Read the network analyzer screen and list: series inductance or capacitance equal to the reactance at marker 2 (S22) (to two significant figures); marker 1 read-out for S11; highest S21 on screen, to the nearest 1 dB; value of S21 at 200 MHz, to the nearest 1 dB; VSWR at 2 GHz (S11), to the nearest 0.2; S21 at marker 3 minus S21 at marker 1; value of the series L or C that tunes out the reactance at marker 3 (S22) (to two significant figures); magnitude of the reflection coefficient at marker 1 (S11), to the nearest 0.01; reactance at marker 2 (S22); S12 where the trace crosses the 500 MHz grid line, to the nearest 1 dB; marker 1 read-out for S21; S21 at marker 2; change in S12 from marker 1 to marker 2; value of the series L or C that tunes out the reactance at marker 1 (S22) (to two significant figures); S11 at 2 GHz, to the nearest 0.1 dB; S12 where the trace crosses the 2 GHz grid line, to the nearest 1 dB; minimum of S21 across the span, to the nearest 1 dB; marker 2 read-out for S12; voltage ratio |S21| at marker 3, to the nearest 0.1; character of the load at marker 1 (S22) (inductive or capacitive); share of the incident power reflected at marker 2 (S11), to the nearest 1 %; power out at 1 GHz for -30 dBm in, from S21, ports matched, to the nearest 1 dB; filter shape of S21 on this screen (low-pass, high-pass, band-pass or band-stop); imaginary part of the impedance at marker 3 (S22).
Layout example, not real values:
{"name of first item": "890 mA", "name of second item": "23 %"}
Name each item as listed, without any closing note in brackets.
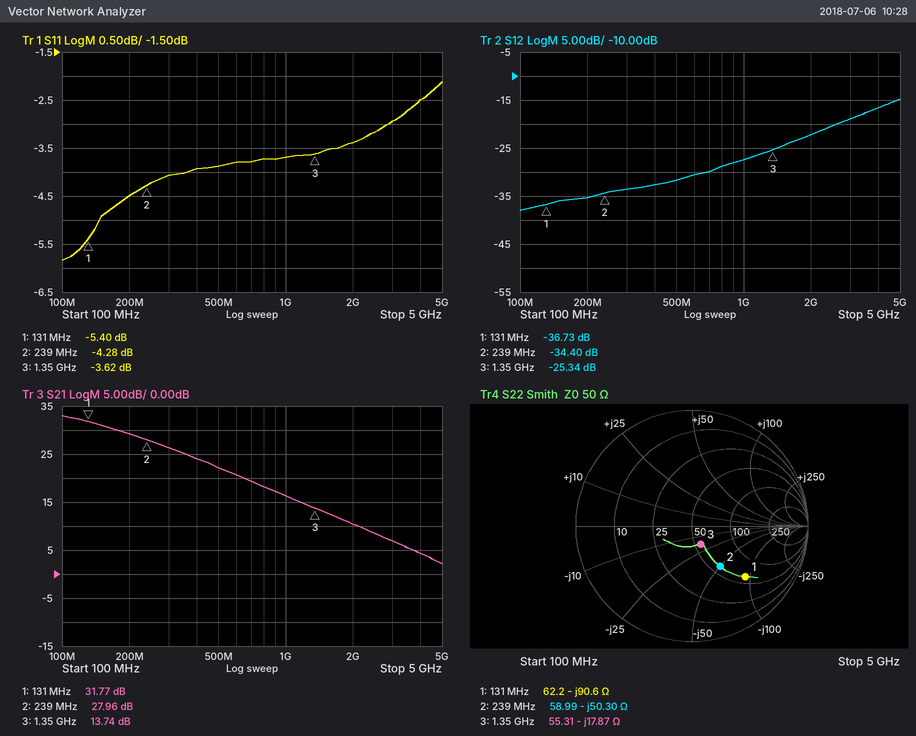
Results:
{"series inductance or capacitance equal to the reactance at marker 2 (S22)": "13 pF", "marker 1 read-out for S11": "-5.40 dB", "highest S21 on screen, to the nearest 1 dB": "33 dB", "value of S21 at 200 MHz, to the nearest 1 dB": "29 dB", "VSWR at 2 GHz (S11), to the nearest 0.2": "5.2", "S21 at marker 3 minus S21 at marker 1": "-18.03 dB", "value of the series L or C that tunes out the reactance at marker 3 (S22)": "2.1 nH", "magnitude of the reflection coefficient at marker 1 (S11), to the nearest 0.01": "0.54", "reactance at marker 2": "-50.30 Ω", "S12 where the trace crosses the 500 MHz grid line, to the nearest 1 dB": "-32 dB", "marker 1 read-out for S21": "31.77 dB", "S21 at marker 2": "27.96 dB", "change in S12 from marker 1 to marker 2": "2.33 dB", "value of the series L or C that tunes out the reactance at marker 1 (S22)": "110 nH", "S11 at 2 GHz, to the nearest 0.1 dB": "-3.4 dB", "S12 where the trace crosses the 2 GHz grid line, to the nearest 1 dB": "-22 dB", "minimum of S21 across the span, to the nearest 1 dB": "2 dB", "marker 2 read-out for S12": "-34.40 dB", "voltage ratio |S21| at marker 3, to the nearest 0.1": "4.9", "character of the load at marker 1 (S22)": "capacitive", "share of the incident power reflected at marker 2 (S11), to the nearest 1 %": "37 %", "power out at 1 GHz for -30 dBm in, from S21, ports matched, to the nearest 1 dB": "-14 dBm", "filter shape of S21 on this screen": "low-pass", "imaginary part of the impedance at marker 3": "-17.87 Ω"}
